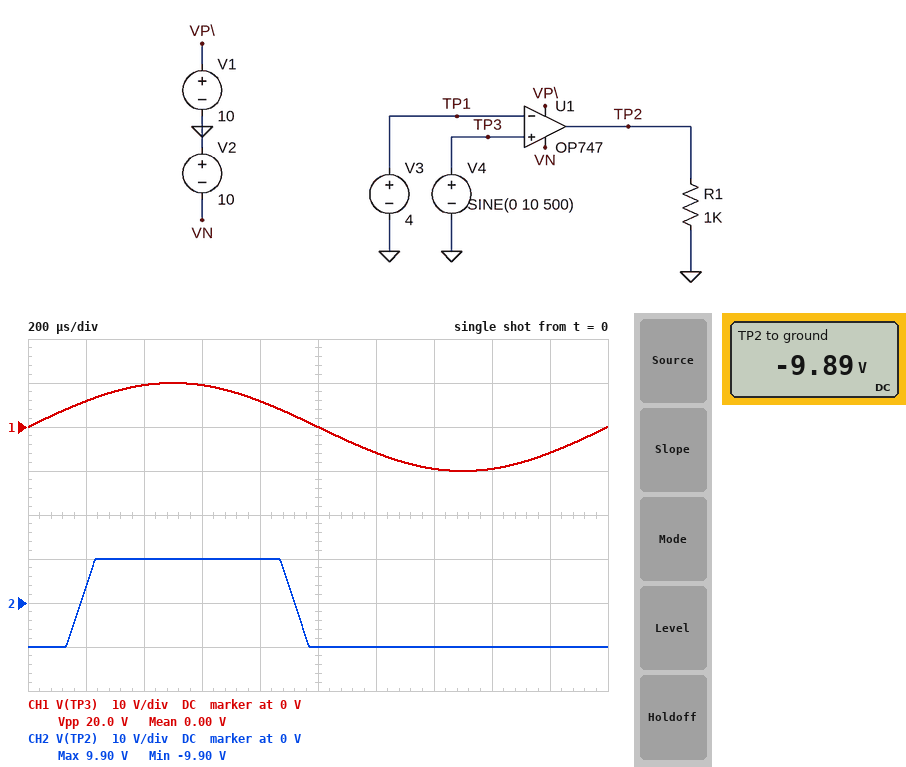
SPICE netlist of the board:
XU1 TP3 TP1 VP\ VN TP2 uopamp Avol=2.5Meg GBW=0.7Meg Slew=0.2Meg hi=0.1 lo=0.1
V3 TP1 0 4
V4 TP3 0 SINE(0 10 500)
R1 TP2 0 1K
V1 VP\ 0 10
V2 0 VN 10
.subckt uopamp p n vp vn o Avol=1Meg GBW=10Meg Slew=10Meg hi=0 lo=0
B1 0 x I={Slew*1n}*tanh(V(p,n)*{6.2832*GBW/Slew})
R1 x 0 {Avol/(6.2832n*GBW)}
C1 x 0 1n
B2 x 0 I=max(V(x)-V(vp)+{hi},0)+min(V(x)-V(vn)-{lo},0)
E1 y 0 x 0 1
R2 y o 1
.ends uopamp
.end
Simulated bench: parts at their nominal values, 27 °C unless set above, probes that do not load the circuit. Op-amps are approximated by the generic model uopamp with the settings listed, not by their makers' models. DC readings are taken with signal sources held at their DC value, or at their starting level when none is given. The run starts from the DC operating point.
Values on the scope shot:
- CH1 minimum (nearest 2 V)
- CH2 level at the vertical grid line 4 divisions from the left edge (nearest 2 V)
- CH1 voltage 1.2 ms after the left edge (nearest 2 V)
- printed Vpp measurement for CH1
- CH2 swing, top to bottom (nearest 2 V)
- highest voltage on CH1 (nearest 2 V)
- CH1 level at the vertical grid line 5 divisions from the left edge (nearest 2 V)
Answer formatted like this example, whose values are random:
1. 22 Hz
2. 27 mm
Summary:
1. -10 V
2. 10 V
3. -6 V
4. 20.0 V
5. 20 V
6. 10 V
7. 0 V
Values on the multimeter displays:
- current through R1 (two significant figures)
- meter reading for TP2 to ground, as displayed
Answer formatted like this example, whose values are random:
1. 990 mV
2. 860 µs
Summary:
1. 9.9 mA
2. -9.89 V
